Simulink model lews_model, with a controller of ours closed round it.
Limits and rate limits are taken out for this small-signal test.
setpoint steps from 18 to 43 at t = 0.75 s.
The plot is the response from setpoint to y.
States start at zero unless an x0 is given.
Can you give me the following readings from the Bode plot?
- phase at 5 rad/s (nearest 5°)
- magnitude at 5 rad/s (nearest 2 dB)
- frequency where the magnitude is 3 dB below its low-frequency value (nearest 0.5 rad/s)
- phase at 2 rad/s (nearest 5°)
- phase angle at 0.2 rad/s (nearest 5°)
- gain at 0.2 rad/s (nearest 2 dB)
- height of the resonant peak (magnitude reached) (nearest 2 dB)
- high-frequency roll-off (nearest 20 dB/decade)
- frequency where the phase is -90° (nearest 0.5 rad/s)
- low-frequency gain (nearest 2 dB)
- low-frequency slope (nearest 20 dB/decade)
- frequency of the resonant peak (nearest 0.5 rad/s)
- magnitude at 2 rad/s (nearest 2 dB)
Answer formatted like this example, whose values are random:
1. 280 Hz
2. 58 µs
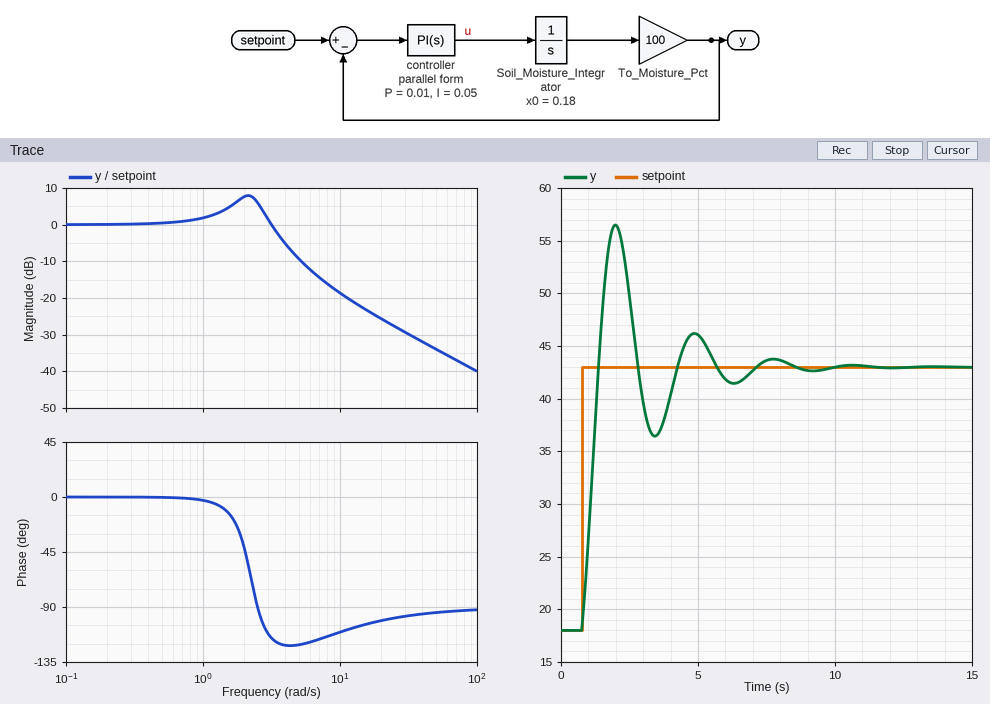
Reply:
1. -120°
2. -10 dB
3. 3.5 rad/s
4. -40°
5. 0°
6. 0 dB
7. 8 dB
8. -20 dB/decade
9. 2.5 rad/s
10. 0 dB
11. 0 dB/decade
12. 2.0 rad/s
13. 8 dB
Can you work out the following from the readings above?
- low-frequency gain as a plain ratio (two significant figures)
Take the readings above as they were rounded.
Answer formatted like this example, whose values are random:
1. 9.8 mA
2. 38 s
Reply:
1. 1.0
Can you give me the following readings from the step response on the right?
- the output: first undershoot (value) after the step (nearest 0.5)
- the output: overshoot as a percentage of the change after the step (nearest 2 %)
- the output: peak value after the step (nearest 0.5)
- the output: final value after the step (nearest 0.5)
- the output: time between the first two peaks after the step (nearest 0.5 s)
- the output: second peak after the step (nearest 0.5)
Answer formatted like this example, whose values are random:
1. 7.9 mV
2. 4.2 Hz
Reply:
1. 36.5
2. 54 %
3. 56.5
4. 43.0
5. 3.0 s
6. 46.0
